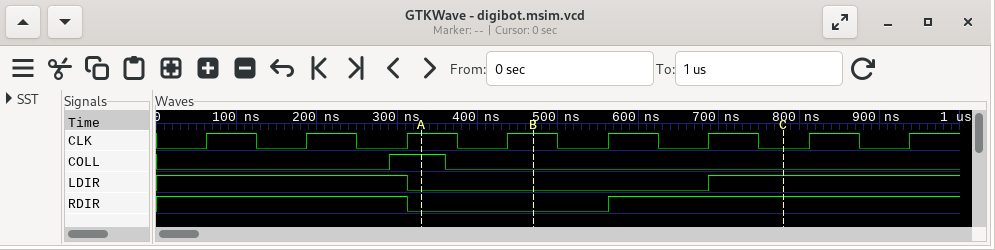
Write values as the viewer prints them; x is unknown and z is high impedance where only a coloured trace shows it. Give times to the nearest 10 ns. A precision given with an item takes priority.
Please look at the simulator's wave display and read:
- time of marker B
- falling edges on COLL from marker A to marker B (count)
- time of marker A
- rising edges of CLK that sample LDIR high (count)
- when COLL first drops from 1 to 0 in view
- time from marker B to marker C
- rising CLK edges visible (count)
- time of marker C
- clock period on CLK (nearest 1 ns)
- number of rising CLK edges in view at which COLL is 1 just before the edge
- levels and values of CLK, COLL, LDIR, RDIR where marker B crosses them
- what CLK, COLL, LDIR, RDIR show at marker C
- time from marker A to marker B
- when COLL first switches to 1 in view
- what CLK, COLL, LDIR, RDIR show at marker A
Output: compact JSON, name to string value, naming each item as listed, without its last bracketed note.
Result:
{"time of marker B": "470 ns", "falling edges on COLL from marker A to marker B": "1", "time of marker A": "330 ns", "rising edges of CLK that sample LDIR high": "5", "when COLL first drops from 1 to 0 in view": "360 ns", "time from marker B to marker C": "310 ns", "rising CLK edges visible": "8", "time of marker C": "780 ns", "clock period on CLK": "125 ns", "number of rising CLK edges in view at which COLL is 1 just before the edge": "1", "levels and values of CLK, COLL, LDIR, RDIR where marker B crosses them": "CLK=1, COLL=0, LDIR=0, RDIR=0", "what CLK, COLL, LDIR, RDIR show at marker C": "CLK=0, COLL=0, LDIR=1, RDIR=1", "time from marker A to marker B": "140 ns", "when COLL first switches to 1 in view": "290 ns", "what CLK, COLL, LDIR, RDIR show at marker A": "CLK=1, COLL=1, LDIR=0, RDIR=0"}
